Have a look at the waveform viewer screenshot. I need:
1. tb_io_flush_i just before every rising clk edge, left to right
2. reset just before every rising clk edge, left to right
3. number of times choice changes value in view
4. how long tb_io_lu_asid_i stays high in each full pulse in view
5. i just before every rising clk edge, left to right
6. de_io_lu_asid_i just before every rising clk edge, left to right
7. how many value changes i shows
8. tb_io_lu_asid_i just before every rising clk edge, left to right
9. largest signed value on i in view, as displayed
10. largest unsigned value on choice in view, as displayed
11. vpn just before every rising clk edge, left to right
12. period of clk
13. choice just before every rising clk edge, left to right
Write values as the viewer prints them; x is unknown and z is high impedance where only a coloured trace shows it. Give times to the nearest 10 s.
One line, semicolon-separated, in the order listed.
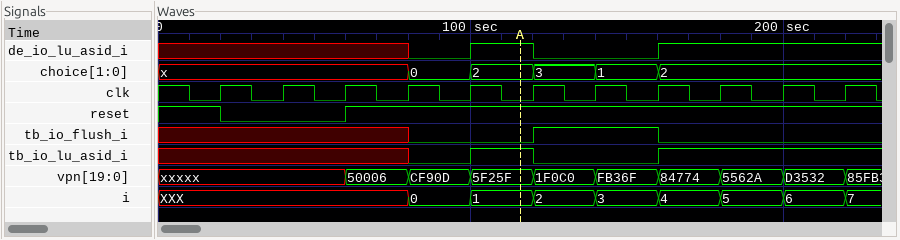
x x x x 0 0 1 1 0 0 0; 1 0 0 1 1 1 1 1 1 1 1; 5; 20 s; XXX, XXX, XXX, XXX, 0, 1, 2, 3, 4, 5, 6; x x x x 0 1 0 0 1 1 1; 8; x x x x 0 1 0 0 1 1 1; 7; 3; xxxxx, xxxxx, xxxxx, 50006, CF90D, 5F25F, 1F0C0, FB36F, 84774, 5562A, D3532; 20 s; x, x, x, x, 0, 2, 3, 1, 2, 2, 2
